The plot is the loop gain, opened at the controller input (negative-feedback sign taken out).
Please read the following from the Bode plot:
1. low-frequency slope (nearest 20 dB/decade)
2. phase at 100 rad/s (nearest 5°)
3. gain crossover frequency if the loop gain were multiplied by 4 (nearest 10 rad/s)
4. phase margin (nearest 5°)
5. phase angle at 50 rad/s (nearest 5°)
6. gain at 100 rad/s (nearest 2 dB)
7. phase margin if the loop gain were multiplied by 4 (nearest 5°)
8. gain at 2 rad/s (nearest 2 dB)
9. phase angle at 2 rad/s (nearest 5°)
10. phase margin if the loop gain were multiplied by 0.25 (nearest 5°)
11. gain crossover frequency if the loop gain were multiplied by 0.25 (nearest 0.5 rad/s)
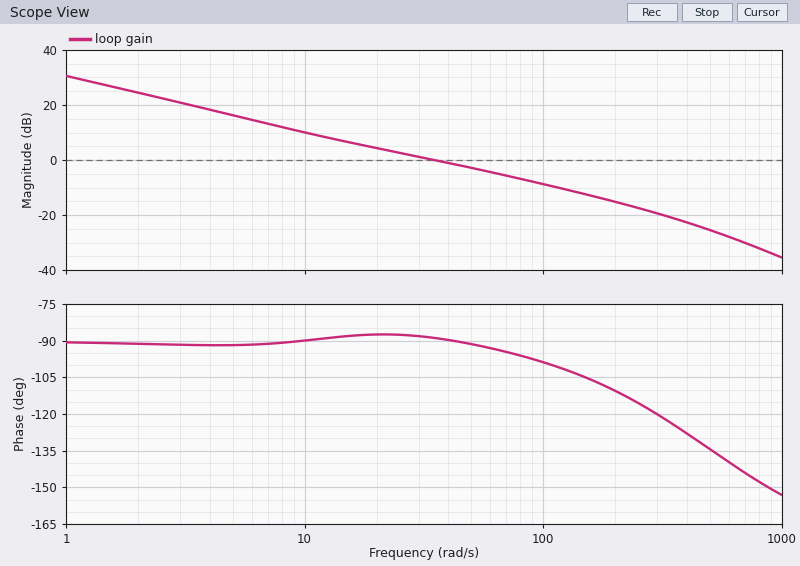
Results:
-20 dB/decade
-100°
140 rad/s
90°
-90°
-8 dB
75°
24 dB
-90°
90°
8.0 rad/s
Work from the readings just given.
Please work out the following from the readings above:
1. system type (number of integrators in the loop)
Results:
1
